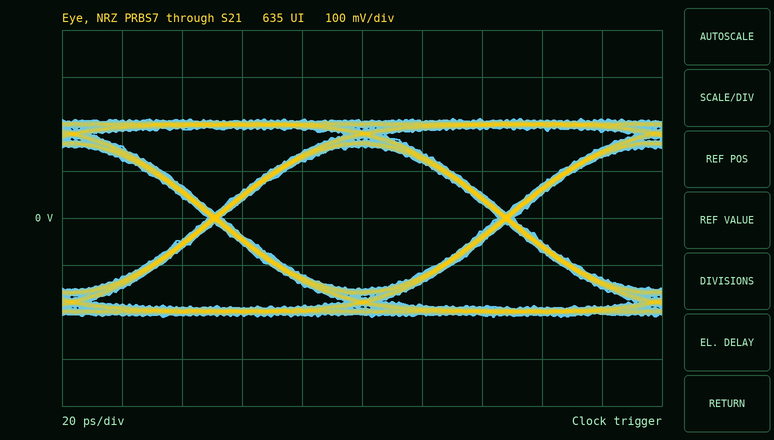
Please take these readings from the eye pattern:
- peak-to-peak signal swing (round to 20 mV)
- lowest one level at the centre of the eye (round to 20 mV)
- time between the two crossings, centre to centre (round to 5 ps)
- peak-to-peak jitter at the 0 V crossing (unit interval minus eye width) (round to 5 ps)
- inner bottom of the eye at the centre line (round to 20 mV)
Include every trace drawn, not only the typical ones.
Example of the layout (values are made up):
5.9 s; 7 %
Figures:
420 mV; 160 mV; 95 ps; 5 ps; -160 mV
